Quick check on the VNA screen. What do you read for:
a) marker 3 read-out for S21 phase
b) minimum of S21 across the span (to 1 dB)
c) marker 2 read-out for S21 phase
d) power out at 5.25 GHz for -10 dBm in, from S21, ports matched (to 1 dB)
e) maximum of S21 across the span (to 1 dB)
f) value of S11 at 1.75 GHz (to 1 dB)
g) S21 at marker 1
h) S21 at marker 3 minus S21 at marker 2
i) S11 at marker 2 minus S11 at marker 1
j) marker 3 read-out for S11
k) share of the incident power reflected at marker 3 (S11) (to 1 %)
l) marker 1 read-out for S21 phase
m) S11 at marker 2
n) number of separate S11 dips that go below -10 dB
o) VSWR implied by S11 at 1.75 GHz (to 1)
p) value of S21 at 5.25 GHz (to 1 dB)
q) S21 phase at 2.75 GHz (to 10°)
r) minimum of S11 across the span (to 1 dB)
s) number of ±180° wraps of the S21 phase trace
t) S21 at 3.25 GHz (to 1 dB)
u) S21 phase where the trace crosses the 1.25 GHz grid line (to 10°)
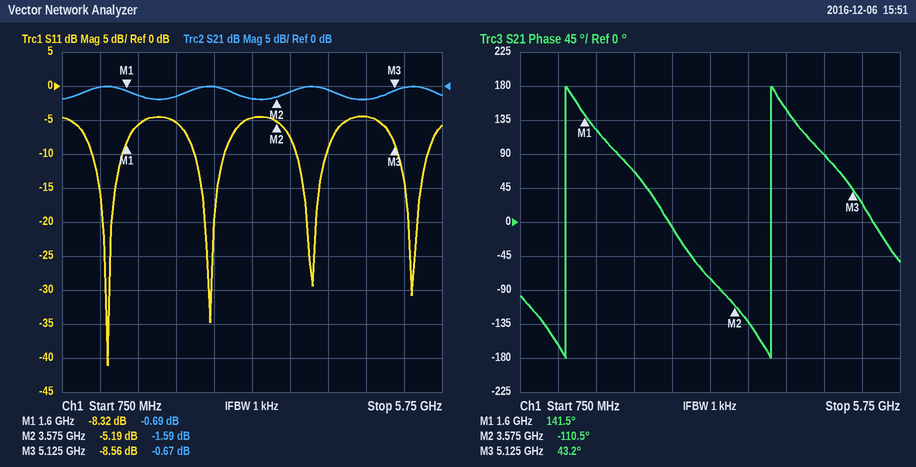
43.2°
-2 dB
-110.5°
-10 dBm
0 dB
-6 dB
-0.69 dB
0.92 dB
3.13 dB
-8.56 dB
14 %
141.5°
-5.19 dB
4
3
0 dB
-10°
-41 dB
2
-2 dB
-160°
